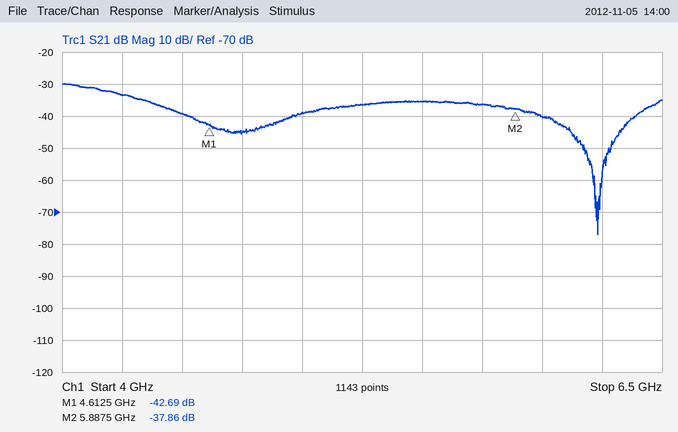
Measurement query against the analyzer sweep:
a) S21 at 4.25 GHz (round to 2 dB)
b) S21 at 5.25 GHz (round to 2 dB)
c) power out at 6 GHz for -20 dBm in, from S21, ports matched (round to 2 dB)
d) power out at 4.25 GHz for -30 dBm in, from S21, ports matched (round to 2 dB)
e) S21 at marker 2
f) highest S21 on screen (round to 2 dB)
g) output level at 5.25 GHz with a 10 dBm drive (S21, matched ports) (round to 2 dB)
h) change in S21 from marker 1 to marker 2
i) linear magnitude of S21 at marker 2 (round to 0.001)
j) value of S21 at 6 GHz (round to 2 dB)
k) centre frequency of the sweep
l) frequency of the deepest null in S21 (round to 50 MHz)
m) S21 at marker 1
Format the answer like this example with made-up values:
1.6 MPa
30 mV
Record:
-34 dB
-36 dB
-60 dBm
-64 dBm
-37.86 dB
-30 dB
-26 dBm
4.83 dB
0.013
-40 dB
5.25 GHz
6.25 GHz
-42.69 dB
